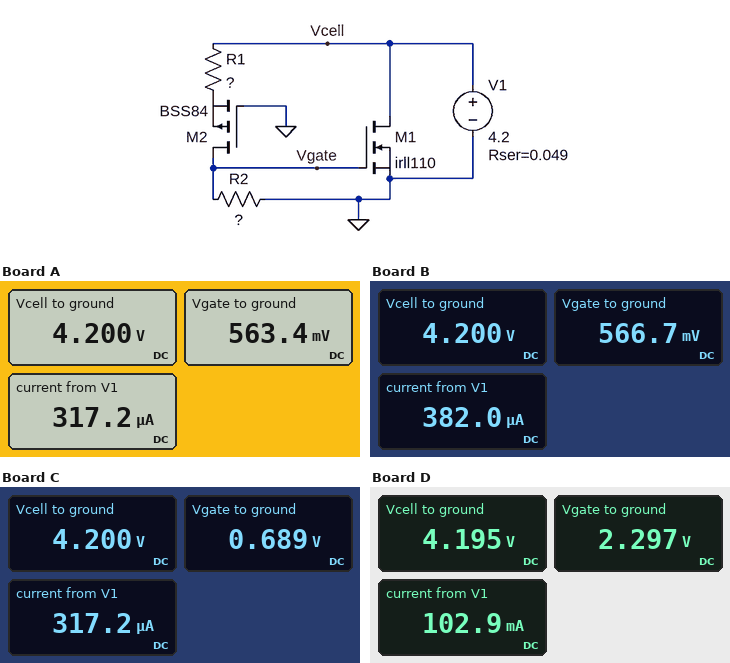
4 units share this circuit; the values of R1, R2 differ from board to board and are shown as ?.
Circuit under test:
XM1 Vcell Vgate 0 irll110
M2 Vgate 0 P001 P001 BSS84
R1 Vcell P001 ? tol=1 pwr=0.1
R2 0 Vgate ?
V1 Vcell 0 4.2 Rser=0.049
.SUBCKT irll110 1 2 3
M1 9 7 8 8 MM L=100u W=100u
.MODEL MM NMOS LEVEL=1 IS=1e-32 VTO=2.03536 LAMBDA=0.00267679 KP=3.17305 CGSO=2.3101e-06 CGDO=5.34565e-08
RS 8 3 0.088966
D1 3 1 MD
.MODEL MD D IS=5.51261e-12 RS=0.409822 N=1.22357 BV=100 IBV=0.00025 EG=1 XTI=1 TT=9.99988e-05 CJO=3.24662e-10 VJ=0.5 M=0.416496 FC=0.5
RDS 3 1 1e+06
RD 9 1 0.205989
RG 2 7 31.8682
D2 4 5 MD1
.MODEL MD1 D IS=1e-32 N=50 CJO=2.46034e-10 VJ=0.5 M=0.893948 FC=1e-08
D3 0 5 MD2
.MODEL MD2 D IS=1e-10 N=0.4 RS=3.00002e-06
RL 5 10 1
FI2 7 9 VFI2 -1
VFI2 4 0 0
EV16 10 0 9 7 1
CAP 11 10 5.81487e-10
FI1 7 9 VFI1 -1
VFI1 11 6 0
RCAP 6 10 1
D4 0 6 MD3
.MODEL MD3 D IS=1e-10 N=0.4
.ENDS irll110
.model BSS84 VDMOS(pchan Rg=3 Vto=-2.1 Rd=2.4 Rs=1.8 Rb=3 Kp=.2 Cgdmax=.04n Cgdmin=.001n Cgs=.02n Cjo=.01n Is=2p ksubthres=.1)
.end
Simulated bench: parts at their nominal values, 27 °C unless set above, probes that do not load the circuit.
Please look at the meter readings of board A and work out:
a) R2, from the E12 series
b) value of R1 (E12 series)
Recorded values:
1.8 kΩ
6.8 kΩ
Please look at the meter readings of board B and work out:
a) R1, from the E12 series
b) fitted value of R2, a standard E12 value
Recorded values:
5.6 kΩ
1.5 kΩ
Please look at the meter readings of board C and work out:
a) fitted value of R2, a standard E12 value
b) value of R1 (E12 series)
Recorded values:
2.2 kΩ
6.8 kΩ
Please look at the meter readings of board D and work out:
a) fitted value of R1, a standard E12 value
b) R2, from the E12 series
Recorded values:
2.7 kΩ
3.3 kΩ
